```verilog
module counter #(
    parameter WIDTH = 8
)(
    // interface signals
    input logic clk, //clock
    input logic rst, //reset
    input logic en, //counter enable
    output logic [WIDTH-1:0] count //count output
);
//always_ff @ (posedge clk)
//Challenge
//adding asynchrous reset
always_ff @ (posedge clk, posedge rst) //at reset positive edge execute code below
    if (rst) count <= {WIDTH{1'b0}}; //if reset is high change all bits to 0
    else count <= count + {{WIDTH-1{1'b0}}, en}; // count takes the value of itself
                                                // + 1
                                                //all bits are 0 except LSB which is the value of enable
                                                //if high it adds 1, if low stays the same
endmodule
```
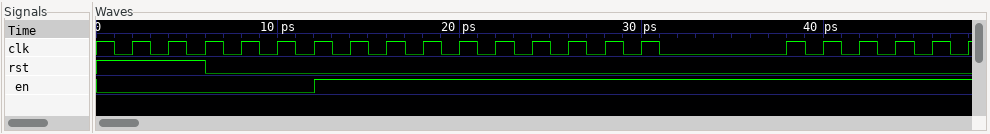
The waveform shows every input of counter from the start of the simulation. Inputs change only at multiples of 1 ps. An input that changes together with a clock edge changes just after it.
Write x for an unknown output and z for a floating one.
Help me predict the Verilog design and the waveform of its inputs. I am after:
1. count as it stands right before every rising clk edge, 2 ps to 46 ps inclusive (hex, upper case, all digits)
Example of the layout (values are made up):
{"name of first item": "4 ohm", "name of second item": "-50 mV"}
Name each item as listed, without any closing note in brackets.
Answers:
{"count as it stands right before every rising clk edge, 2 ps to 46 ps inclusive": "00, 00, 00, 00, 00, 00, 00, 01, 02, 03, 04, 05, 06, 07, 08, 09, 0A, 0B, 0C, 0D"}
